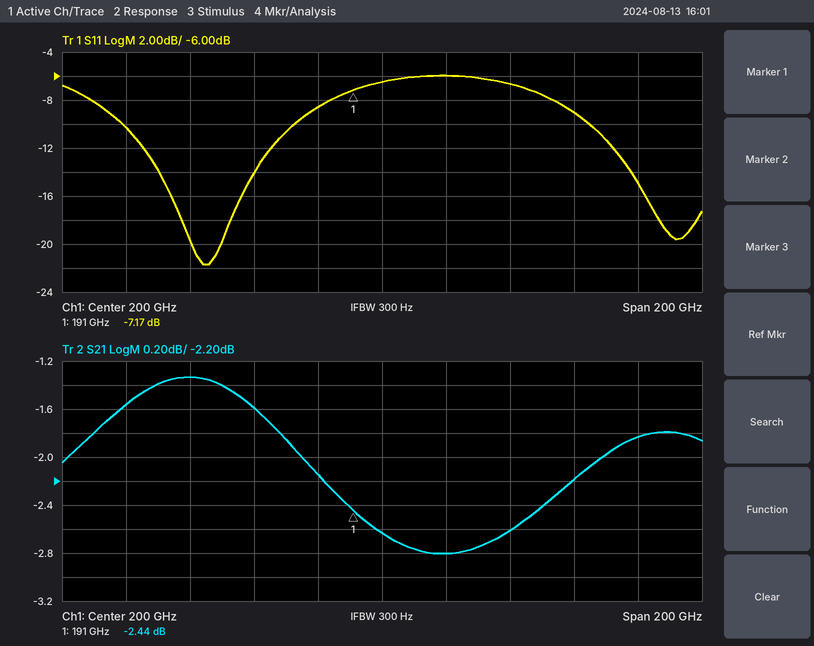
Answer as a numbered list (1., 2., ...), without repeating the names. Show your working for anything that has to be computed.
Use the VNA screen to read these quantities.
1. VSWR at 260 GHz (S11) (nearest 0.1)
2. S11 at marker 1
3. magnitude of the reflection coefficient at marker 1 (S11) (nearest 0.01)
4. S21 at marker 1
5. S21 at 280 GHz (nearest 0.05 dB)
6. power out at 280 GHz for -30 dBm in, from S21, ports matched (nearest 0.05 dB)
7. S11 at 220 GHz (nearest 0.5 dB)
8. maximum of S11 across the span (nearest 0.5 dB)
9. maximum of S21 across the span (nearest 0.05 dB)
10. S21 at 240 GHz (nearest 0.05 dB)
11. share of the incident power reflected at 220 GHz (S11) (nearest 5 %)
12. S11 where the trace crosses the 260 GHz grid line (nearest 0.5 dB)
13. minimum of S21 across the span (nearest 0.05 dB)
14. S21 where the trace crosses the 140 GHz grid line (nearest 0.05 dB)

1. |Γ| = 10^(-9/20) = 0.3548; VSWR = (1 + 0.3548)/(1 − 0.3548) ≈ 2.1
2. -7.17 dB
3. 10^(-7.17/20) ≈ 0.44
4. -2.44 dB
5. -1.85 dB
6. -30 dBm + (-1.85 dB) = -31.85 dBm
7. -6.0 dB
8. -6.0 dB
9. -1.35 dB
10. -2.60 dB
11. 10^(-6/10) ≈ 25 %
12. -9.0 dB
13. -2.80 dB
14. -1.35 dB
